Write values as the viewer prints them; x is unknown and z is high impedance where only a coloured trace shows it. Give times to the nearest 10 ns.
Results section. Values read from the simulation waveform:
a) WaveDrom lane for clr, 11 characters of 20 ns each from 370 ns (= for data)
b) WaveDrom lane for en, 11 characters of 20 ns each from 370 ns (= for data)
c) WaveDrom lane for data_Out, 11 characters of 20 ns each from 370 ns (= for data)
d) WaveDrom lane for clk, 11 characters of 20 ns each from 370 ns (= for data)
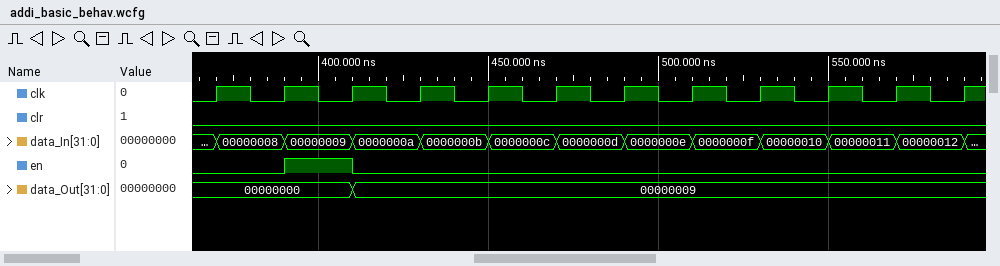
{name: 'clr', wave: '0..........'}
{name: 'en', wave: '010........'}
{name: 'data_Out', wave: '=.=........', data: '00000000 00000009'}
{name: 'clk', wave: 'p..........'}
